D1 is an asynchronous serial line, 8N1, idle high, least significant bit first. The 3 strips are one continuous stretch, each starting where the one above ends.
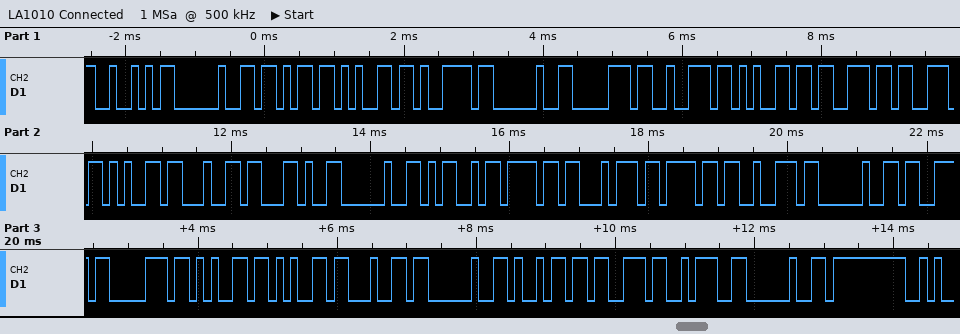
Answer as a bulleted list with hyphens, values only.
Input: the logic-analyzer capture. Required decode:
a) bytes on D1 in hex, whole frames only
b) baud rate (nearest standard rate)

- 52 20 6B 65 79 20 70 72 65 73 73 65 64 2C 20 4D 6F 74 6F 72 20 73 70 65 65 64 20 69 73 3A 20 FF
- 9600 baud
